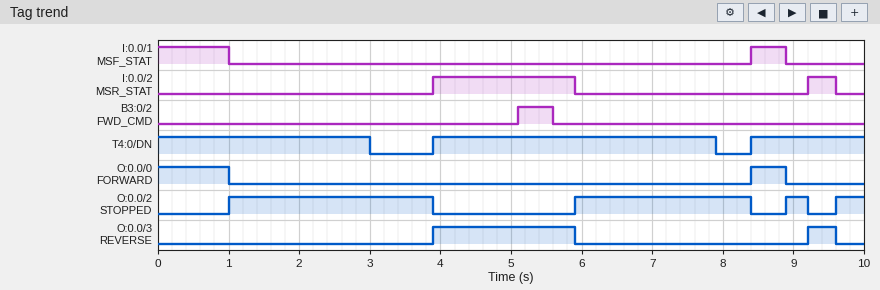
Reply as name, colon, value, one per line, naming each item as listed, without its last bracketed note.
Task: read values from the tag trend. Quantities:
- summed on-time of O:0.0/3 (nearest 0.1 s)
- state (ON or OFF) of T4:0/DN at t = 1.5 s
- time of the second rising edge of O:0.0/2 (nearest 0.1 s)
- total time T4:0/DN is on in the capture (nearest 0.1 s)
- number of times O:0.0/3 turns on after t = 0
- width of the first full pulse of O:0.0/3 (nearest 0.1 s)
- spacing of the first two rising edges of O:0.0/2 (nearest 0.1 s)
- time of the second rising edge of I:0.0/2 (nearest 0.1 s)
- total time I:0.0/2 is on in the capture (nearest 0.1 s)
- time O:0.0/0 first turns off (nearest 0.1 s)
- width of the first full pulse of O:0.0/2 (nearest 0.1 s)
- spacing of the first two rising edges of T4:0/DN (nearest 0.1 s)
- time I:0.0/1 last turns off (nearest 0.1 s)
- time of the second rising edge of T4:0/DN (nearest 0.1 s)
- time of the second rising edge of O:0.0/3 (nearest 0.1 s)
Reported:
summed on-time of O:0.0/3: 2.4 s
state (ON or OFF) of T4:0/DN at t = 1.5 s: ON
time of the second rising edge of O:0.0/2: 5.9 s
total time T4:0/DN is on in the capture: 8.6 s
number of times O:0.0/3 turns on after t = 0: 2
width of the first full pulse of O:0.0/3: 2.0 s
spacing of the first two rising edges of O:0.0/2: 4.9 s
time of the second rising edge of I:0.0/2: 9.2 s
total time I:0.0/2 is on in the capture: 2.4 s
time O:0.0/0 first turns off: 1.0 s
width of the first full pulse of O:0.0/2: 2.9 s
spacing of the first two rising edges of T4:0/DN: 4.5 s
time I:0.0/1 last turns off: 8.9 s
time of the second rising edge of T4:0/DN: 8.4 s
time of the second rising edge of O:0.0/3: 9.2 s
